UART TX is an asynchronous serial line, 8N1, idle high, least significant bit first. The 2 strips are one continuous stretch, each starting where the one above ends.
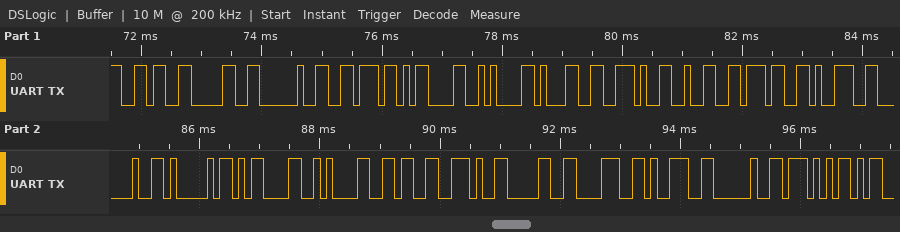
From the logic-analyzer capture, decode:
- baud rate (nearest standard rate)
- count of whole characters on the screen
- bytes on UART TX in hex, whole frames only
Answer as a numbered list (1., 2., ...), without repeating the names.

1. 9600 baud
2. 22
3. 36 30 20 76 0D 0A 31 2E 32 37 39 20 41 0D 0A 36 2E 30 38 39 20 57
